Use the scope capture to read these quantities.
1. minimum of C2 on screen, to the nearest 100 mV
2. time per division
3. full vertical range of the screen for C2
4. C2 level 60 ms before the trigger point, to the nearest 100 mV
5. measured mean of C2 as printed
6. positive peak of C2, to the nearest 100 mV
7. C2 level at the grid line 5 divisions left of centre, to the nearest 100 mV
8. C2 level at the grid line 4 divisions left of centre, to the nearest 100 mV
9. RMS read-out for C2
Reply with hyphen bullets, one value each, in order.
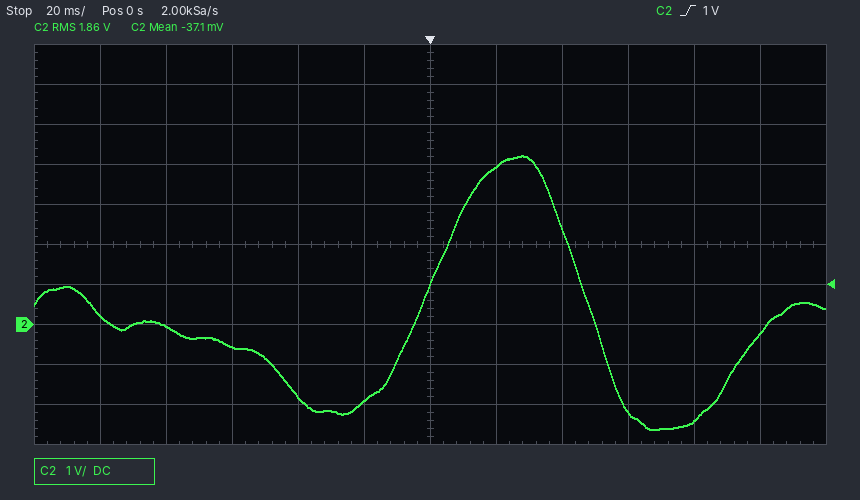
- -2.6 V
- 20 ms
- 10 V
- -600 mV
- -37.1 mV
- 4.2 V
- 200 mV
- 0.0 V
- 1.86 V
